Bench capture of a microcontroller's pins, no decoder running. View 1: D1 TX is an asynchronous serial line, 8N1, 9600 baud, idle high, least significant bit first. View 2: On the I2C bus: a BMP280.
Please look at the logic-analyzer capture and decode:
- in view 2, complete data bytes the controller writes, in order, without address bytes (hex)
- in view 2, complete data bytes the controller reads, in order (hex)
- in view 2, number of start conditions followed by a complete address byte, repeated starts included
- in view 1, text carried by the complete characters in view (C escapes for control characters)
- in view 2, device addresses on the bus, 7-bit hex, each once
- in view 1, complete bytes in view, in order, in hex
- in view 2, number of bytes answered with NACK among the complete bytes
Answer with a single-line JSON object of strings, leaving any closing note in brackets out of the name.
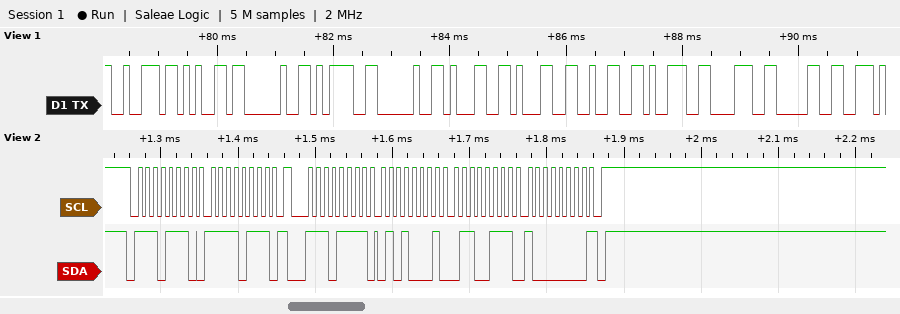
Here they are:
{"in view 2, complete data bytes the controller writes, in order, without address bytes": "F7", "in view 2, complete data bytes the controller reads, in order": "51 67 80", "in view 2, number of start conditions followed by a complete address byte, repeated starts included": "2", "in view 1, text carried by the complete characters in view": "\"re = 112980\"", "in view 2, device addresses on the bus, 7-bit hex, each once": "0x77", "in view 1, complete bytes in view, in order, in hex": "0x72 0x65 0x20 0x3D 0x20 0x31 0x31 0x32 0x39 0x38 0x30", "in view 2, number of bytes answered with NACK among the complete bytes": "1"}
